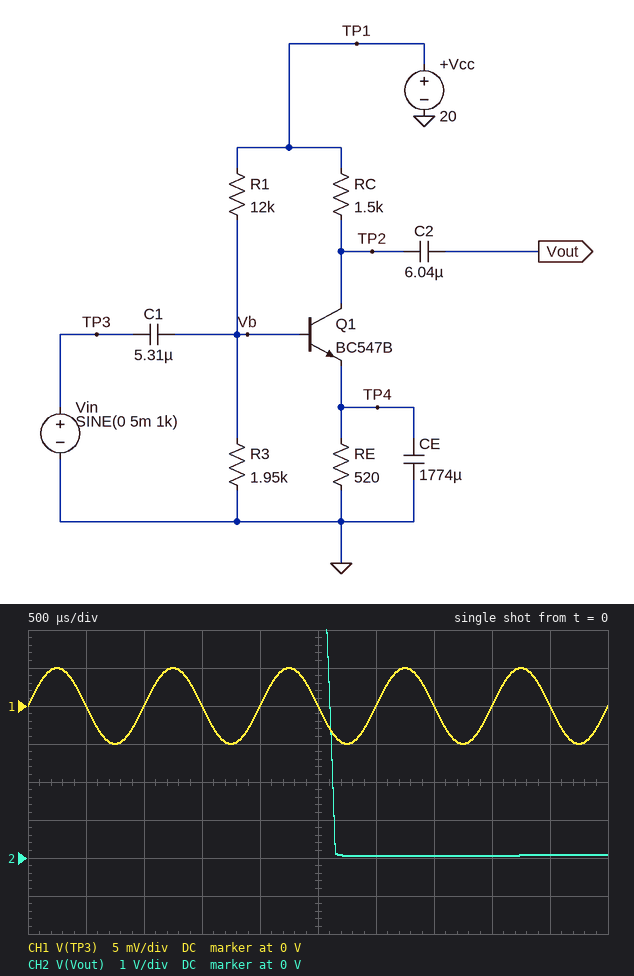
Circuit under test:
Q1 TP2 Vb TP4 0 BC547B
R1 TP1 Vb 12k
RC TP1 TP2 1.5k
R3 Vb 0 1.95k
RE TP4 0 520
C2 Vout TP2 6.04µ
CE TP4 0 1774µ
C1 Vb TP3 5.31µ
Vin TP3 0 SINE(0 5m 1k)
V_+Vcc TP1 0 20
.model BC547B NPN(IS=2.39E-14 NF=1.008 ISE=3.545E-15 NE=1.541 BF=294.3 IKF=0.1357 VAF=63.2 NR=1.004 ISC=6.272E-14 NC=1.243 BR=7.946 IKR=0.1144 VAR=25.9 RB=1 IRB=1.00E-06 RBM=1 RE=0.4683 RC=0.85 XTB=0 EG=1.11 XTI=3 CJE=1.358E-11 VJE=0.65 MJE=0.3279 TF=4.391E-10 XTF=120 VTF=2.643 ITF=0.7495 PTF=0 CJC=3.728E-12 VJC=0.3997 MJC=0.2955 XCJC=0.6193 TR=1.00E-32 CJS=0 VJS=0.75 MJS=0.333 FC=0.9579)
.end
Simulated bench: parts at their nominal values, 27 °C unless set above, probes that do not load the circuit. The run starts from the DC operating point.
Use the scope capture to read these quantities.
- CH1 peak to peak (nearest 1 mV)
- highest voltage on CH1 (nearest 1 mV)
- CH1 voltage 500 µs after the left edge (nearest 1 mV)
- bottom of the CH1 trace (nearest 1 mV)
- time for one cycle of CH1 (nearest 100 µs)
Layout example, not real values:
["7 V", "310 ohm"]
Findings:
["10 mV", "5 mV", "0 V", "-5 mV", "1.0 ms"]
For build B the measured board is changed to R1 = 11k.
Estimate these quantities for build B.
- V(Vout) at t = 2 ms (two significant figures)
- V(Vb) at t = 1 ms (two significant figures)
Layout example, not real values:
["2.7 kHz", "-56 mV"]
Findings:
["19 V", "330 mV"]
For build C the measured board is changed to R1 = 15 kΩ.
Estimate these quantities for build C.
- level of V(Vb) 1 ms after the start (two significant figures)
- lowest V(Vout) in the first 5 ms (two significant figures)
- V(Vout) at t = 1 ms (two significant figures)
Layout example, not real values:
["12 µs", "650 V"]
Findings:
["240 mV", "61 mV", "20 V"]
